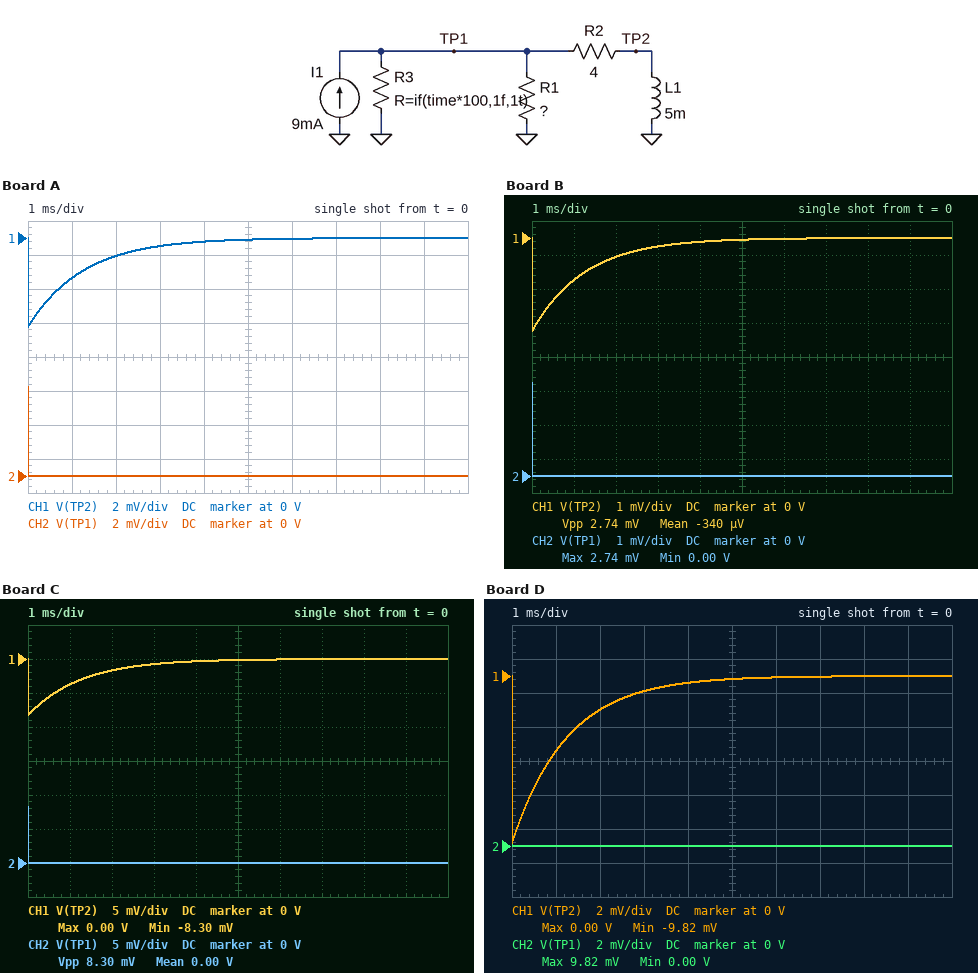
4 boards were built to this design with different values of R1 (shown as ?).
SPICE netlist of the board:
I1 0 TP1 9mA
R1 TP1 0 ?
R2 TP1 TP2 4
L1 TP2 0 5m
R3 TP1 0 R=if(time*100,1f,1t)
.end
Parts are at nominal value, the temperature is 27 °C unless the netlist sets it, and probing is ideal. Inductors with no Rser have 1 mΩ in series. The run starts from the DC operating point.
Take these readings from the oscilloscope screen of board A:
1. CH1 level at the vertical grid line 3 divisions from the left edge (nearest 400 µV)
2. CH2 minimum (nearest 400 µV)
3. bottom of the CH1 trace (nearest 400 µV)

-400 µV
0 V
-5.2 mV
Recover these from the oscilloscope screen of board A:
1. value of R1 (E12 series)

0.68 Ω
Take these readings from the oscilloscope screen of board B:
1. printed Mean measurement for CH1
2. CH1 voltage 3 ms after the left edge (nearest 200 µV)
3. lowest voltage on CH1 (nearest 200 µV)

-340 µV
-200 µV
-2.8 mV
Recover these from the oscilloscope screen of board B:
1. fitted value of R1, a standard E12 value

0.33 Ω
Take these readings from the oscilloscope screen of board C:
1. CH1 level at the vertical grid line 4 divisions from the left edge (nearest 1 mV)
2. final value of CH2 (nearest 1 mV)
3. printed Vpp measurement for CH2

0 V
0 V
8.30 mV
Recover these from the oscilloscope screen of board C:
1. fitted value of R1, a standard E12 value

1.2 Ω
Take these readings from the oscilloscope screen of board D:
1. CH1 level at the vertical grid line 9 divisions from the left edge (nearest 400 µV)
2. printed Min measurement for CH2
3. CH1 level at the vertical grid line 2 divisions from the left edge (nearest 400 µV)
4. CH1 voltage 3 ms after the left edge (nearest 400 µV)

0 V
0.00 V
-2.0 mV
-800 µV
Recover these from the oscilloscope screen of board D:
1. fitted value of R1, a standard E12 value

1.5 Ω
